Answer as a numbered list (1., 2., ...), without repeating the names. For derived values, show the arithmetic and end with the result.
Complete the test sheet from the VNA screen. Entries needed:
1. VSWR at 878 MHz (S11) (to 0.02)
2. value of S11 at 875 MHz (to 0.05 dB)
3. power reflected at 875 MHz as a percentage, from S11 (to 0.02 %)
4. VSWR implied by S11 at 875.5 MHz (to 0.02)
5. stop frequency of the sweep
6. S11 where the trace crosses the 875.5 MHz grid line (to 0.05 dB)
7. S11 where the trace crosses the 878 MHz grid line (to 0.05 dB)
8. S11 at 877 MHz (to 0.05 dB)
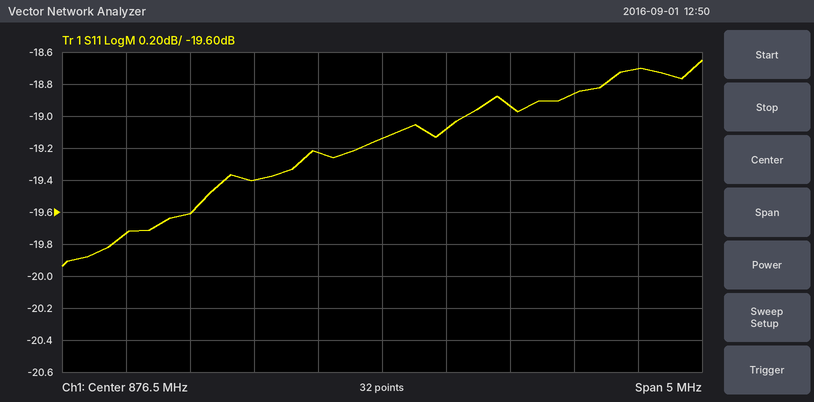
1. |Γ| = 10^(-18.85/20) = 0.1142; VSWR = (1 + 0.1142)/(1 − 0.1142) ≈ 1.26
2. -19.60 dB
3. 10^(-19.6/10) ≈ 1.10 %
4. |Γ| = 10^(-19.4/20) = 0.1072; VSWR = (1 + 0.1072)/(1 − 0.1072) ≈ 1.24
5. 879 MHz
6. -19.40 dB
7. -18.85 dB
8. -19.10 dB
